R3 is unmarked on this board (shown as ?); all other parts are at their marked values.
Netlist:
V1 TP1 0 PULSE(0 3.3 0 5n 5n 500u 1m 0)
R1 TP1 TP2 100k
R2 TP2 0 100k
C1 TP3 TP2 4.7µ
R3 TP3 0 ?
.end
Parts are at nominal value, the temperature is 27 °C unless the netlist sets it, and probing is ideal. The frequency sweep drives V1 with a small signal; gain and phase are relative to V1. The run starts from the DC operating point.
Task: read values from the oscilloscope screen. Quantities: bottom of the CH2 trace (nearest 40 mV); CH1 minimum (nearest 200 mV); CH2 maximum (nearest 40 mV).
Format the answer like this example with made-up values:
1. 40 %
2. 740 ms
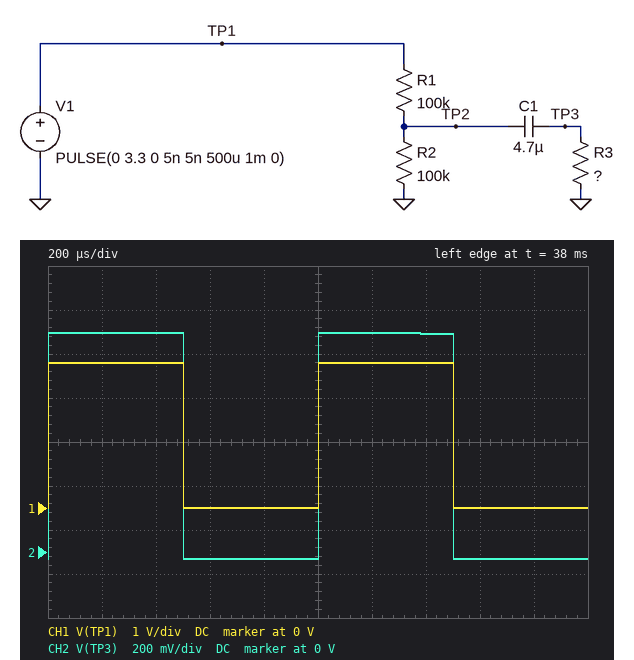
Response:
1. -40 mV
2. 0 V
3. 1.00 V
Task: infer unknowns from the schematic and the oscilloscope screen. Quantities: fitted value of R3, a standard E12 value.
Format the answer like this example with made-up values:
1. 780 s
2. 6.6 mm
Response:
1. 82 kΩ
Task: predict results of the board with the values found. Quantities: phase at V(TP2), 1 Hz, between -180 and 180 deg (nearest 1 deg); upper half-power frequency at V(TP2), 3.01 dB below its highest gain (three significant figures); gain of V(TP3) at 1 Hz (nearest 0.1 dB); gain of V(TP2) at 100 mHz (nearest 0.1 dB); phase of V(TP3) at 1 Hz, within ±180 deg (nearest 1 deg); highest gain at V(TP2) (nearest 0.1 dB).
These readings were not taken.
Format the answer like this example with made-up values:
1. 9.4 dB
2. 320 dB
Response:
1. -8 deg
2. 537 mHz
3. -10.4 dB
4. -6.4 dB
5. 14 deg
6. -6.0 dB
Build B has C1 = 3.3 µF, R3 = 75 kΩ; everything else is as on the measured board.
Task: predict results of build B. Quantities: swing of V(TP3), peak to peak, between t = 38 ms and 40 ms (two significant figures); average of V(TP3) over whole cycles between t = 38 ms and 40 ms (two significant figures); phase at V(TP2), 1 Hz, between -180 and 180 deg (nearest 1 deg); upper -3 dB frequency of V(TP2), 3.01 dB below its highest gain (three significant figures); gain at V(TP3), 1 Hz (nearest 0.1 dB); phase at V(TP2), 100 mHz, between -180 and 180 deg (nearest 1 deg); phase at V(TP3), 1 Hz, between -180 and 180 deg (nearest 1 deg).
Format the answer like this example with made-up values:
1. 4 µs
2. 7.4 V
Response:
1. 990 mV
2. 450 mV
3. -12 deg
4. 729 mHz
5. -11.1 dB
6. -6 deg
7. 21 deg
